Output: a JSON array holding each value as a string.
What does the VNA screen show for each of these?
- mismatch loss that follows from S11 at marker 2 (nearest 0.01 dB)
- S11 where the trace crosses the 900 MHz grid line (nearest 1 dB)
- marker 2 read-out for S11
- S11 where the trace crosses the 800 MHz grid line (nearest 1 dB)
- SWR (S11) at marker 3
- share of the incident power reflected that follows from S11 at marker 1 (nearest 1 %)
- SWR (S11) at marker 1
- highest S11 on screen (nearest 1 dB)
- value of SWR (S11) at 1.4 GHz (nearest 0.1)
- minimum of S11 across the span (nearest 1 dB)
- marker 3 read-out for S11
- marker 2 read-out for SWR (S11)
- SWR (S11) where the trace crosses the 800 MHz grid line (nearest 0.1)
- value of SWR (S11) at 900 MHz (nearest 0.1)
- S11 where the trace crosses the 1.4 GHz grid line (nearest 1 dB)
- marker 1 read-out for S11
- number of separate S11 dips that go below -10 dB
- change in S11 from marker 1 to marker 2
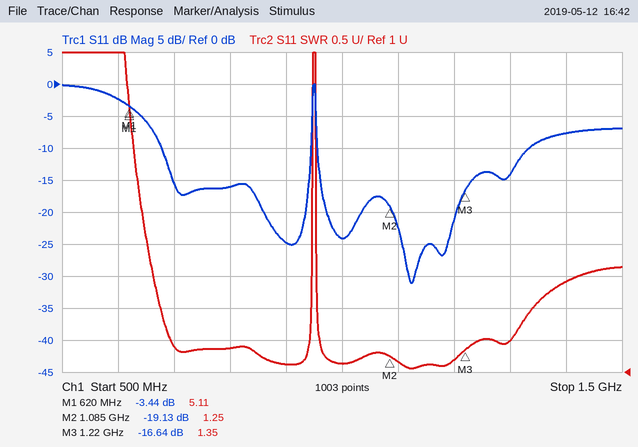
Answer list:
["0.05 dB", "-25 dB", "-19.13 dB", "-16 dB", "1.35", "45 %", "5.11", "0 dB", "2.4", "-31 dB", "-16.64 dB", "1.25", "1.4", "1.1", "-8 dB", "-3.44 dB", "3", "-15.69 dB"]
